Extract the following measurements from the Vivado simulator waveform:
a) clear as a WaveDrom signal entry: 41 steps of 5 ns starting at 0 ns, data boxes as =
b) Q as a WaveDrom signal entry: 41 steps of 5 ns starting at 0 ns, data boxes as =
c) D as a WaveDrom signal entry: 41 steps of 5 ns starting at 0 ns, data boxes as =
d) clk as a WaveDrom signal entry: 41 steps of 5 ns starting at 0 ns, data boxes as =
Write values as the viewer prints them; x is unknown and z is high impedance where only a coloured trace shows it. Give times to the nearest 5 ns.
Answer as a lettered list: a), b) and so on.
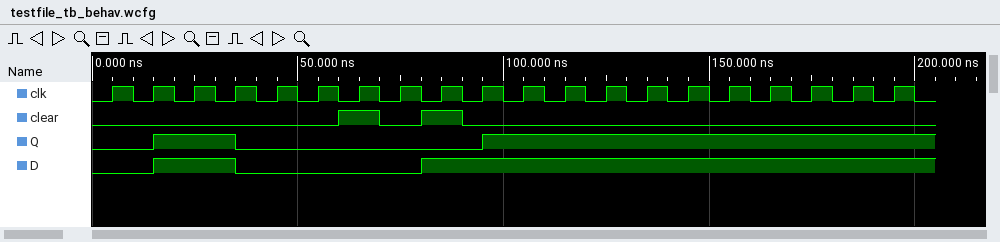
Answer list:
a) {name: 'clear', wave: '0...........1.0.1.0......................'}
b) {name: 'Q', wave: '0..1...0...........1.....................'}
c) {name: 'D', wave: '0..1...0........1........................'}
d) {name: 'clk', wave: '01010101010101010101010101010101010101010'}
